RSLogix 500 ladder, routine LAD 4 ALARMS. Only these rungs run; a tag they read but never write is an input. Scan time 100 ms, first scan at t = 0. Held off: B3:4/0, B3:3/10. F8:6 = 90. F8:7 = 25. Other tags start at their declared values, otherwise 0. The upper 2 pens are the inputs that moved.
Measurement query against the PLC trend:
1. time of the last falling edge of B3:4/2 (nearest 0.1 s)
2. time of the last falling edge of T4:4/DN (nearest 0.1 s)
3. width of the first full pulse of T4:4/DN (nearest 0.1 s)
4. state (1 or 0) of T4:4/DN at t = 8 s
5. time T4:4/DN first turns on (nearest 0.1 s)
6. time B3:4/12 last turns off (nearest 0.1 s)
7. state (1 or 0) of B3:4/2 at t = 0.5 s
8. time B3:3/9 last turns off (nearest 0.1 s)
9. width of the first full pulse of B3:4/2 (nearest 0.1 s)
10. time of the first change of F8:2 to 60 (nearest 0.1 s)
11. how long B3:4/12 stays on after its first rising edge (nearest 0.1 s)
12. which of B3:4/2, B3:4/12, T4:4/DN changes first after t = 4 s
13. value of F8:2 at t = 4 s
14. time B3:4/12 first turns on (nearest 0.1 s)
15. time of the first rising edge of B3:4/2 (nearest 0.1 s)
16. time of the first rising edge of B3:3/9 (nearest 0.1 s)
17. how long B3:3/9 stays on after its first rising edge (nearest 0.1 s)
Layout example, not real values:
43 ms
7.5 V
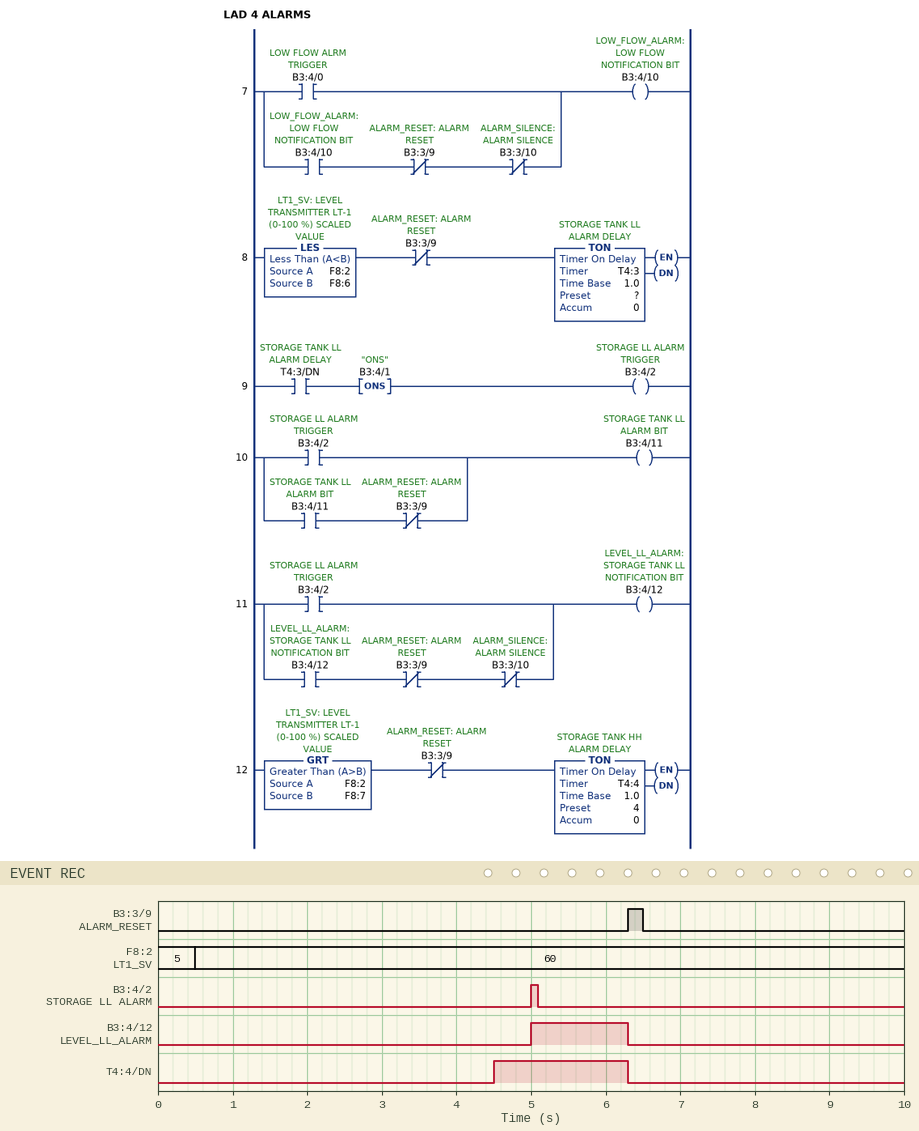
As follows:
5.1 s
6.3 s
1.8 s
0
4.5 s
6.3 s
0
6.5 s
0.1 s
0.5 s
1.3 s
T4:4/DN
60
5.0 s
5.0 s
6.3 s
0.2 s
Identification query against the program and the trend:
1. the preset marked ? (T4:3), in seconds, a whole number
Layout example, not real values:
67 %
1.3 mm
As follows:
5 s
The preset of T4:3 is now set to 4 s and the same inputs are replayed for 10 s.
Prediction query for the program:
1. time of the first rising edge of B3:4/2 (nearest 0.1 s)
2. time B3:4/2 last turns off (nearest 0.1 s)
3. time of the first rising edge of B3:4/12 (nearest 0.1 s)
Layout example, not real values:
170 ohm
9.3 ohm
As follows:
4.0 s
4.1 s
4.0 s
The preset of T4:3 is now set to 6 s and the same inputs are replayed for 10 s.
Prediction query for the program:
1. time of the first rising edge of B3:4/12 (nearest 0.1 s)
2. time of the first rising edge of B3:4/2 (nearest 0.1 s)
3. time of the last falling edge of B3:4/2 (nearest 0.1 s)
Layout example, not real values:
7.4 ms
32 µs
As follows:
6.0 s
6.0 s
6.1 s
